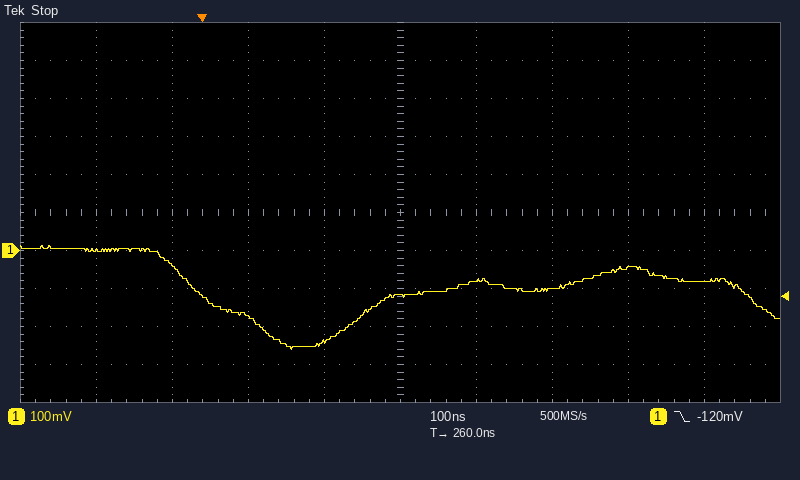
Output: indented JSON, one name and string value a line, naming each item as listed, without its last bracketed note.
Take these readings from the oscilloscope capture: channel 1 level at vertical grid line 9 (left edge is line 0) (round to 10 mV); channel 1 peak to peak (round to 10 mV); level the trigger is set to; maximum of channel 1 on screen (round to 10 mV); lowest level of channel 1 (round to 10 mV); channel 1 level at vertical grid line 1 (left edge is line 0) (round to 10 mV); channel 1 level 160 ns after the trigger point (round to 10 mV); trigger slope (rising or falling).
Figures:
{
  "channel 1 level at vertical grid line 9 (left edge is line 0)": "-80 mV",
  "channel 1 peak to peak": "270 mV",
  "level the trigger is set to": "-120 mV",
  "maximum of channel 1 on screen": "10 mV",
  "lowest level of channel 1": "-260 mV",
  "channel 1 level at vertical grid line 1 (left edge is line 0)": "0 mV",
  "channel 1 level 160 ns after the trigger point": "-240 mV",
  "trigger slope": "falling"
}
